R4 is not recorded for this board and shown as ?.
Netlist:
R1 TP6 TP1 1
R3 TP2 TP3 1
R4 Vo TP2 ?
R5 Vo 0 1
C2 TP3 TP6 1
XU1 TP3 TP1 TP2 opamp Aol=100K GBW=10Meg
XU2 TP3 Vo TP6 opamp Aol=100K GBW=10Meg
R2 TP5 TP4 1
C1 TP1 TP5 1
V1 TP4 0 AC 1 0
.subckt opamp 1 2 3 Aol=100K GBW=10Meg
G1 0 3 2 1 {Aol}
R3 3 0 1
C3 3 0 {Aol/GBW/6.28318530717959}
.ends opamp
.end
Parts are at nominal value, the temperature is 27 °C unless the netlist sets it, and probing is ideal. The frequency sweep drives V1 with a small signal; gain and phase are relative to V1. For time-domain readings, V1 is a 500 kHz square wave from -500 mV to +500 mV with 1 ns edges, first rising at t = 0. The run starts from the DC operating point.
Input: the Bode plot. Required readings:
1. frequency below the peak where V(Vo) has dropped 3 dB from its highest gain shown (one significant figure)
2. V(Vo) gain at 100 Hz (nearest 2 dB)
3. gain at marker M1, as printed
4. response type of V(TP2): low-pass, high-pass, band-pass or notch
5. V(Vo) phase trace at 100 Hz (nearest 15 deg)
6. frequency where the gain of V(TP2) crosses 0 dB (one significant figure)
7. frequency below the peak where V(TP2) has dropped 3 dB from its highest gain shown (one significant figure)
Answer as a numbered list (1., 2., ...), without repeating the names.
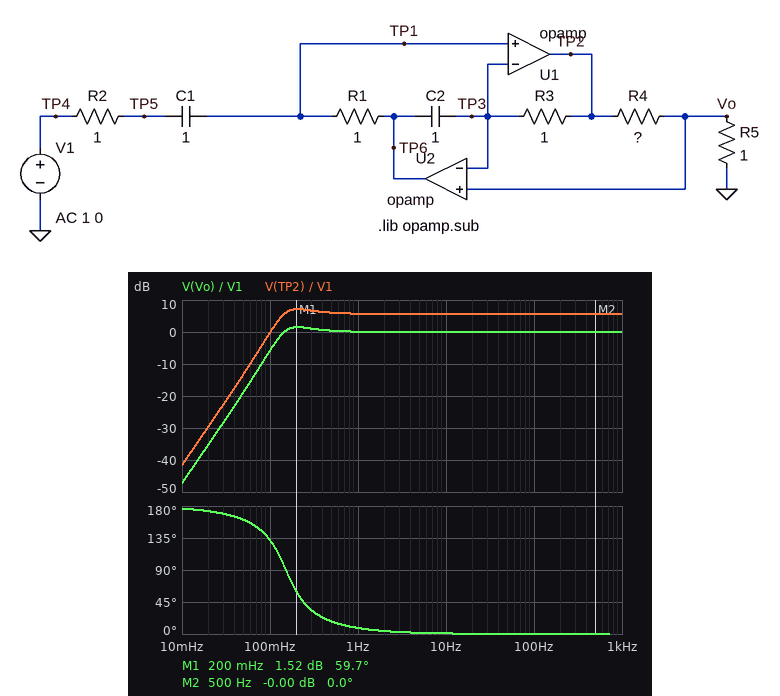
1. 100 mHz
2. 0 dB
3. 1.52 dB
4. high-pass
5. 0 deg
6. 100 mHz
7. 100 mHz
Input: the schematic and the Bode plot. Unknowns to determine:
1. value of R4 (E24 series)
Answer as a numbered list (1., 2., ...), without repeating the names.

1. 0.91 Ω
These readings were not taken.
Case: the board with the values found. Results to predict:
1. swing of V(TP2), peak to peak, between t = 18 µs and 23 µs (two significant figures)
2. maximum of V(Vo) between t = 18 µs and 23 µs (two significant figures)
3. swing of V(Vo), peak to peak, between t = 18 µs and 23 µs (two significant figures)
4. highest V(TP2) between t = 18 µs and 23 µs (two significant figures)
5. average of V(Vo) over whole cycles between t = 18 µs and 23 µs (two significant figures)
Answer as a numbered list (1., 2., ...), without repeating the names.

1. 1.9 V
2. 1.0 V
3. 1.0 V
4. 1.9 V
5. 500 mV
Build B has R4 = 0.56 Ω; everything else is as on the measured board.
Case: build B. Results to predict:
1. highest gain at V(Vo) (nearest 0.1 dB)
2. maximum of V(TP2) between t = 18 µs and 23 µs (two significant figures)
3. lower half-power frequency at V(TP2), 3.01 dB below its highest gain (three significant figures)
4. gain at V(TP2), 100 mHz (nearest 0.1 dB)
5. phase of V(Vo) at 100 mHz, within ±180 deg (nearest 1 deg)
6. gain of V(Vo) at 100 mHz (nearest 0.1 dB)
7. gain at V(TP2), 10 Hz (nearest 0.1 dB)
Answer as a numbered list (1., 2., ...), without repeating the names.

1. 3.2 dB
2. 1.6 V
3. 100 mHz
4. 4.0 dB
5. 115 deg
6. 0.1 dB
7. 3.9 dB
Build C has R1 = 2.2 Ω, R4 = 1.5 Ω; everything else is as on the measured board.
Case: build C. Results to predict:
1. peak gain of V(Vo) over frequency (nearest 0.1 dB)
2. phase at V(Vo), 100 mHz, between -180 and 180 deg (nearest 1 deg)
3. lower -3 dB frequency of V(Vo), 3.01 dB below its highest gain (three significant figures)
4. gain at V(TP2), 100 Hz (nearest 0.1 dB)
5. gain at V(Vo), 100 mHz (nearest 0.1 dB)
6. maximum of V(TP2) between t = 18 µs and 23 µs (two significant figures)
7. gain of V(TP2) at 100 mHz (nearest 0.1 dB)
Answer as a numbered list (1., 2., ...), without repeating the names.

1. 2.5 dB
2. 124 deg
3. 111 mHz
4. 8.0 dB
5. -2.3 dB
6. 2.5 V
7. 5.6 dB
